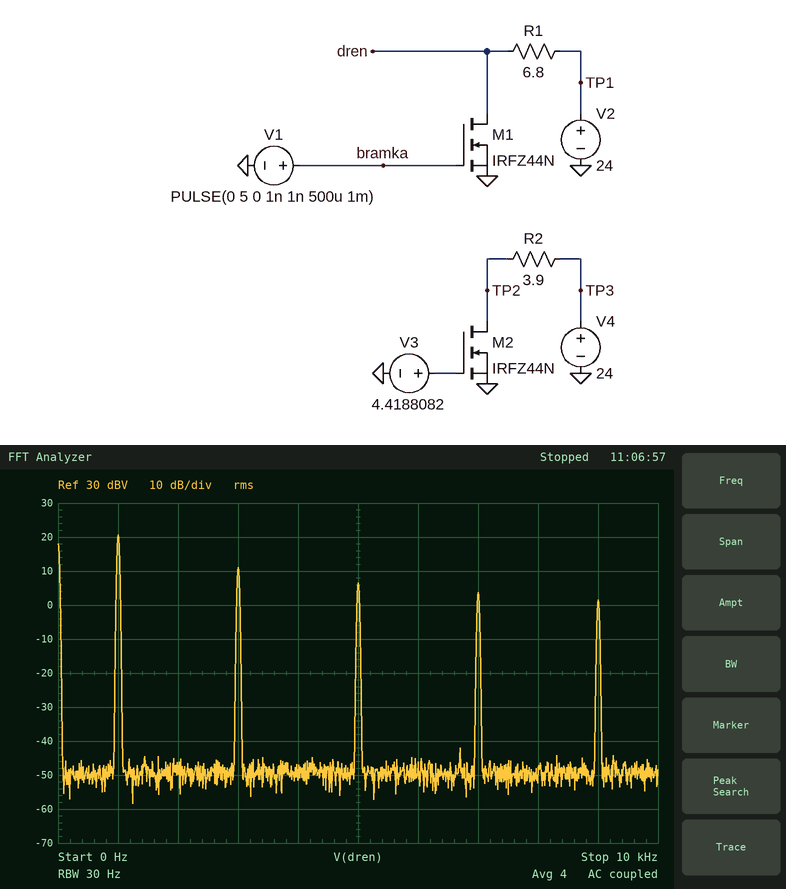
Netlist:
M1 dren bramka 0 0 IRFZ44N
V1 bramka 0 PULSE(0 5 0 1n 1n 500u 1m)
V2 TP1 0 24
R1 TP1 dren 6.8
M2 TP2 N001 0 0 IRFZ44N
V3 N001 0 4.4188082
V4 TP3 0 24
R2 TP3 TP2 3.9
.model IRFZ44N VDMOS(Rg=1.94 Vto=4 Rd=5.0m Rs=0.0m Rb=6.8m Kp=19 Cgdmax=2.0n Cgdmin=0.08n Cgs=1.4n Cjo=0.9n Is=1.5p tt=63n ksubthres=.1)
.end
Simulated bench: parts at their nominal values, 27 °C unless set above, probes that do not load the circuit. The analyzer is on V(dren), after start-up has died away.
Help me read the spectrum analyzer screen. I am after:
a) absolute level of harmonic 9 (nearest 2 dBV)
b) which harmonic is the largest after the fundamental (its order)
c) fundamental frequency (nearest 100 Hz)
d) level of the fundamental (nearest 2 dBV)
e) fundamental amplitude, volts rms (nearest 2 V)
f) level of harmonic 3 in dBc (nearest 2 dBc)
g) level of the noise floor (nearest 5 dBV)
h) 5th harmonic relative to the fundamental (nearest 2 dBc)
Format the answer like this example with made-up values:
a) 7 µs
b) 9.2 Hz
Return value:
a) 2 dBV
b) 3
c) 1.0 kHz
d) 20 dBV
e) 10 V
f) -10 dBc
g) -50 dBV
h) -14 dBc
